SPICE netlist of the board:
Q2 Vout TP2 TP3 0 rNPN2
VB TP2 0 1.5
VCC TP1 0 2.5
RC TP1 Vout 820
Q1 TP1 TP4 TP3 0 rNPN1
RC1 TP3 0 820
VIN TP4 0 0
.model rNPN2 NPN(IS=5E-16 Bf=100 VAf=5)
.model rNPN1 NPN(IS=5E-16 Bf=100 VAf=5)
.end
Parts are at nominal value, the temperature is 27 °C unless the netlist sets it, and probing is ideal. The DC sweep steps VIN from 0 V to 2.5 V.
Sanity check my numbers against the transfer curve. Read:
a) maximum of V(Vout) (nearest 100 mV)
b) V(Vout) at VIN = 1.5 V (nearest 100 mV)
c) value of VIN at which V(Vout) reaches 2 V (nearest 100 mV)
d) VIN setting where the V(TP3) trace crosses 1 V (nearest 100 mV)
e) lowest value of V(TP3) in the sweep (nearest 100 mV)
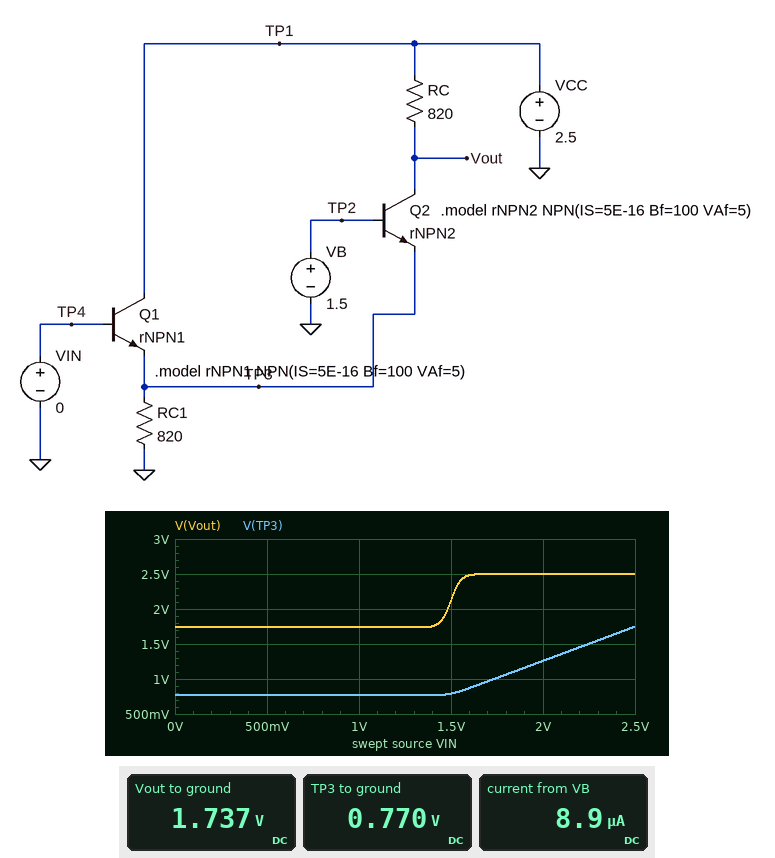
2.5 V
2.1 V
1.5 V
1.7 V
800 mV
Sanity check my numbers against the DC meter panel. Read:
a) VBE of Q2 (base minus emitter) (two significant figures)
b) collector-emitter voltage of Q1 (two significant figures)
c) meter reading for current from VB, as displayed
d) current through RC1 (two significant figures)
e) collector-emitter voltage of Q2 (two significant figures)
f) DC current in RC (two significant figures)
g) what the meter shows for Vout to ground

730 mV
1.7 V
8.9 µA
940 µA
970 mV
930 µA
1.737 V
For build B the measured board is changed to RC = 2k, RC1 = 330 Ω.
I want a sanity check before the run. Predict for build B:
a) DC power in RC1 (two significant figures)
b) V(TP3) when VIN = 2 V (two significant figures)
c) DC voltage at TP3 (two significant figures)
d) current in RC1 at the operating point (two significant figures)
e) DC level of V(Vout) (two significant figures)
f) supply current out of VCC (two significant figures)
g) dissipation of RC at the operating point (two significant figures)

1.6 mW
1.2 V
730 mV
2.2 mA
760 mV
870 µA
1.5 mW
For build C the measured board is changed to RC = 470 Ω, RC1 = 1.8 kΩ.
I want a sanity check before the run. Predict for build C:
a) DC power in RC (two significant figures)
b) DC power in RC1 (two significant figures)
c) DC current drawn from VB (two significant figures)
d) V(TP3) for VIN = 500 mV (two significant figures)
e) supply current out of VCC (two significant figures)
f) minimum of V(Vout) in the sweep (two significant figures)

90 µW
350 µW
3.8 µA
790 mV
440 µA
2.3 V
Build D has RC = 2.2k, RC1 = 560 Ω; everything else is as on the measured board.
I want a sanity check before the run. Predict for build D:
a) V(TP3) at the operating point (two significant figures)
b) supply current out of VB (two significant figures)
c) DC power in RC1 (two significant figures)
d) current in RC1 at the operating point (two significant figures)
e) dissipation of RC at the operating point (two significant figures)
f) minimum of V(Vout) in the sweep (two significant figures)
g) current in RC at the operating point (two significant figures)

750 mV
560 µA
1.0 mW
1.3 mA
1.3 mW
780 mV
780 µA
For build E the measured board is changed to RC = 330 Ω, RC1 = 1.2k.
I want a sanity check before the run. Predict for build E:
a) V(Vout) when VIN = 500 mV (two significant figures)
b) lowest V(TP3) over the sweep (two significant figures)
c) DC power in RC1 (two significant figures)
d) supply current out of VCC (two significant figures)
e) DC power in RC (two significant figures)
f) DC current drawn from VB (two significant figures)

2.3 V
780 mV
510 µW
650 µA
140 µW
5.6 µA
